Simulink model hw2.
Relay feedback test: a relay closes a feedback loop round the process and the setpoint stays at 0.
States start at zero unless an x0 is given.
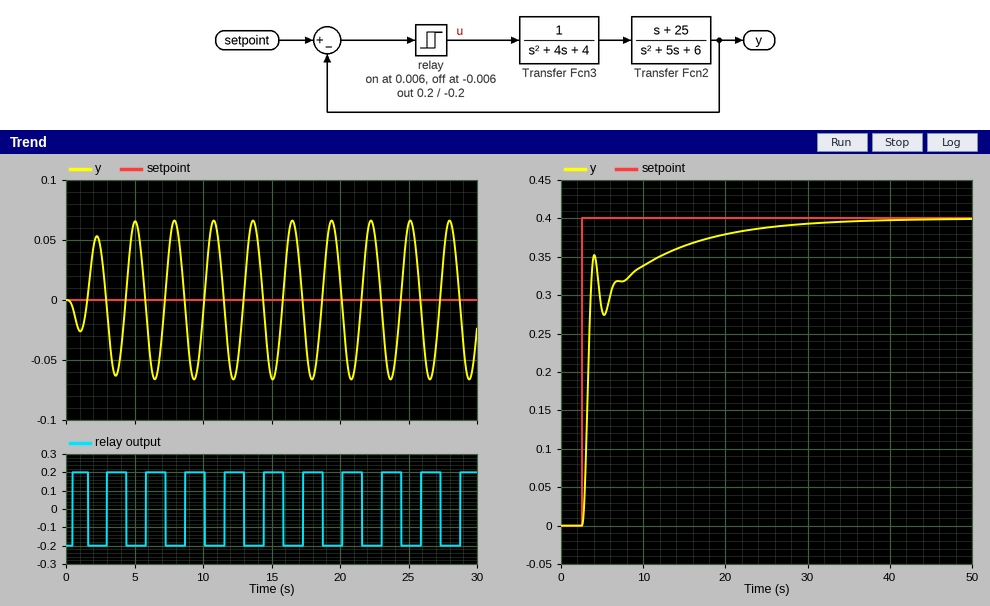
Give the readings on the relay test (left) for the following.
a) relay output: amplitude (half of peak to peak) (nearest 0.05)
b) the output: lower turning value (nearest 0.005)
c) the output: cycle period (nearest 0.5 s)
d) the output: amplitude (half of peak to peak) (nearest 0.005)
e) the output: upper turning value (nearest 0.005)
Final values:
0.20
-0.065
3.0 s
0.065
0.065
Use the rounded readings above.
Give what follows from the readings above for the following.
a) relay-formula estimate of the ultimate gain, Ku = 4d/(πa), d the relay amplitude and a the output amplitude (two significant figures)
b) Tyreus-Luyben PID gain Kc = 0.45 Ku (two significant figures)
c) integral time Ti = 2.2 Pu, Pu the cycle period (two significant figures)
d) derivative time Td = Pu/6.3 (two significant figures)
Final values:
3.9
1.8
6.6 s
0.48 s
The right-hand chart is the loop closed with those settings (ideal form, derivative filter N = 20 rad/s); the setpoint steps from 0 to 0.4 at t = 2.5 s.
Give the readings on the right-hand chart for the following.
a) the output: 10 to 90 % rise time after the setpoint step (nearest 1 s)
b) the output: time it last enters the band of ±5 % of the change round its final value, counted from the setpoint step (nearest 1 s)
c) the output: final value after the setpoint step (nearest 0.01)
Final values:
11 s
18 s
0.40
